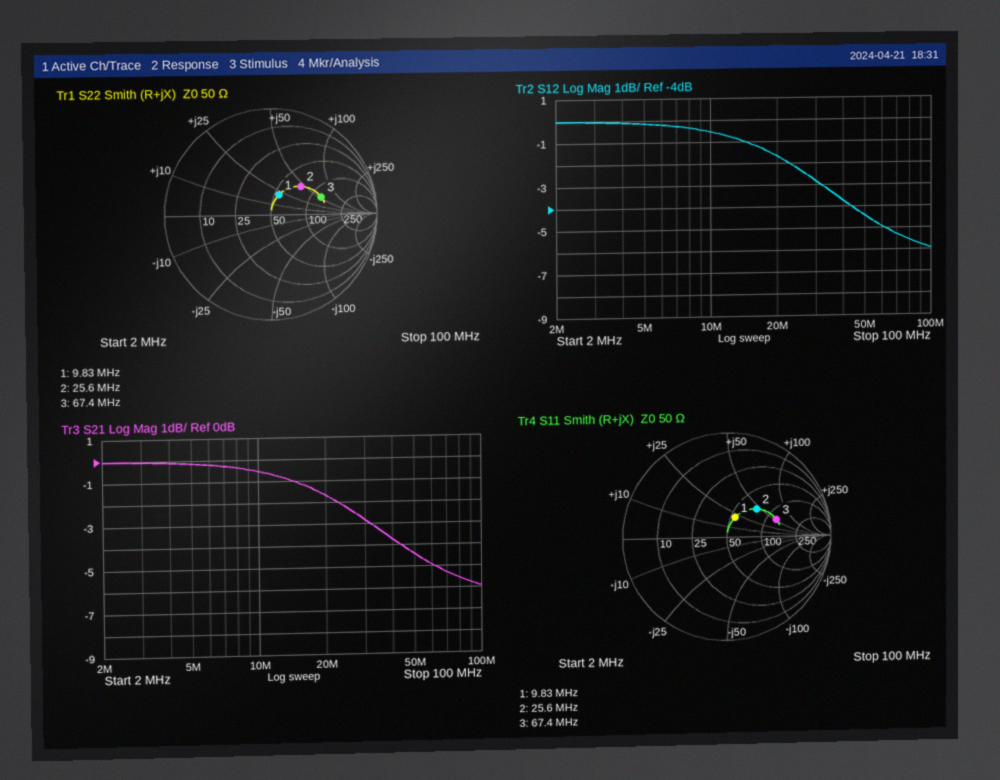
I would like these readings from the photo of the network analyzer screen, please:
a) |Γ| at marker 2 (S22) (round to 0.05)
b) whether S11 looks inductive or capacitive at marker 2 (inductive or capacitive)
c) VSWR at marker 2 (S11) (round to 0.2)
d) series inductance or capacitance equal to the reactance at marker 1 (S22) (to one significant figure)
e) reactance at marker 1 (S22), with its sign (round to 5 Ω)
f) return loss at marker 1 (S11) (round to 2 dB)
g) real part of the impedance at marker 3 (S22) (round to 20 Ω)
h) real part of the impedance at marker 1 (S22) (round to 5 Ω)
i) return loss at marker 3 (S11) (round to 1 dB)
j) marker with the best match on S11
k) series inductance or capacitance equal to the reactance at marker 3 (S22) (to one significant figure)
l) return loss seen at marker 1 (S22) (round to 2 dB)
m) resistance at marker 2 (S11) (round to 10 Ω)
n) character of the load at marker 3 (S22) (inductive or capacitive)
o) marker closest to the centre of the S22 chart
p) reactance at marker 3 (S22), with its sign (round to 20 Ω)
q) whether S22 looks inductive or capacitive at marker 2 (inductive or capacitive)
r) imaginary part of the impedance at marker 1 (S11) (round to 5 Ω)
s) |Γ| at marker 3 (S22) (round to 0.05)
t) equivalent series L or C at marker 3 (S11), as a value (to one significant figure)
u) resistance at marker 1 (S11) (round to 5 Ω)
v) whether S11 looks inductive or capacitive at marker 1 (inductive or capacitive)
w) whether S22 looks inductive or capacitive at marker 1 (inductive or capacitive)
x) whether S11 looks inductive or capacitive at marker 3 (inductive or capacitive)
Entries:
0.40
inductive
2.2
300 nH
+20 Ω
14 dB
120 Ω
55 Ω
6 dB
marker 1
100 nH
14 dB
70 Ω
inductive
marker 1
+60 Ω
inductive
+20 Ω
0.50
100 nH
55 Ω
inductive
inductive
inductive
